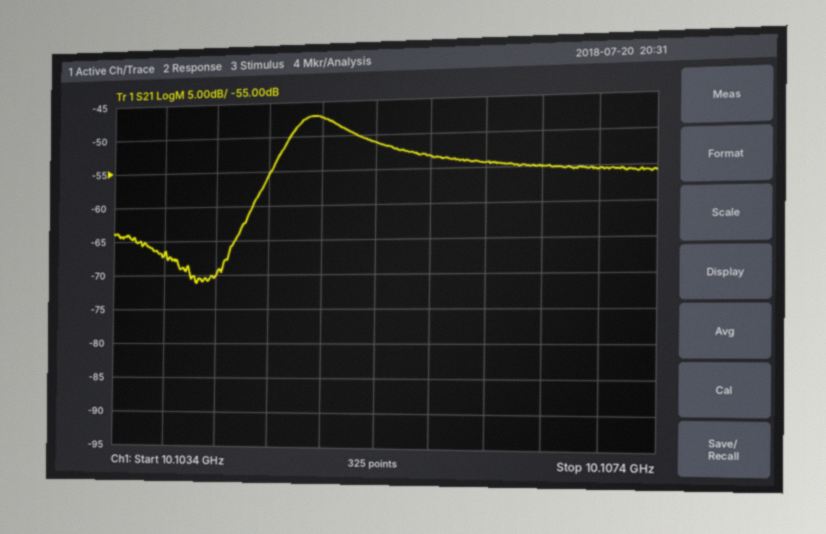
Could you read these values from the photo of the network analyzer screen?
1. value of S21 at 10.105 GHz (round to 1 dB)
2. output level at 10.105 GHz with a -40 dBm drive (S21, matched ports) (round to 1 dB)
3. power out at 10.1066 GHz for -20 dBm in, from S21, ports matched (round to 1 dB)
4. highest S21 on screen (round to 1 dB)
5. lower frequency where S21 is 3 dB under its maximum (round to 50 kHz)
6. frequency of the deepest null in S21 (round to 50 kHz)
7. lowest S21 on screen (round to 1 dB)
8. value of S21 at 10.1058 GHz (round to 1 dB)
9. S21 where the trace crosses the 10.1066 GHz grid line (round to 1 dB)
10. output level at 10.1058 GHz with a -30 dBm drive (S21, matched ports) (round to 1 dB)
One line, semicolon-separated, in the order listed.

-47 dB; -87 dBm; -75 dBm; -47 dB; 10.10475 GHz; 10.10405 GHz; -71 dB; -53 dB; -55 dB; -83 dBm
